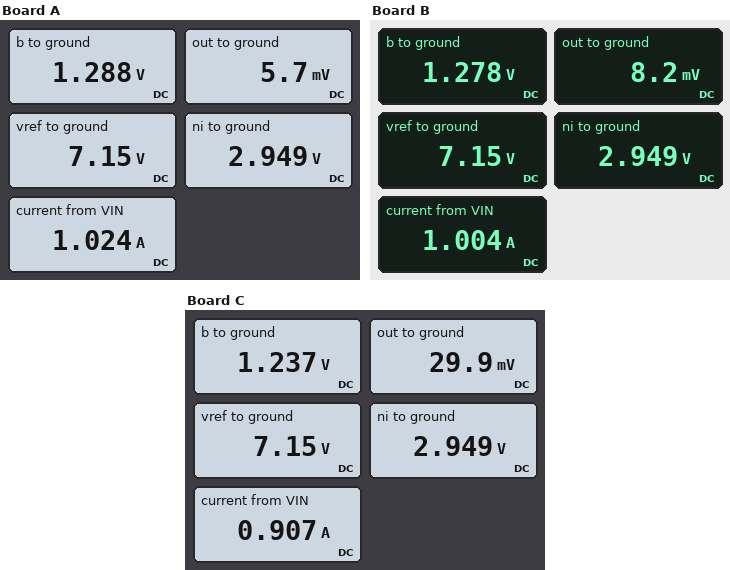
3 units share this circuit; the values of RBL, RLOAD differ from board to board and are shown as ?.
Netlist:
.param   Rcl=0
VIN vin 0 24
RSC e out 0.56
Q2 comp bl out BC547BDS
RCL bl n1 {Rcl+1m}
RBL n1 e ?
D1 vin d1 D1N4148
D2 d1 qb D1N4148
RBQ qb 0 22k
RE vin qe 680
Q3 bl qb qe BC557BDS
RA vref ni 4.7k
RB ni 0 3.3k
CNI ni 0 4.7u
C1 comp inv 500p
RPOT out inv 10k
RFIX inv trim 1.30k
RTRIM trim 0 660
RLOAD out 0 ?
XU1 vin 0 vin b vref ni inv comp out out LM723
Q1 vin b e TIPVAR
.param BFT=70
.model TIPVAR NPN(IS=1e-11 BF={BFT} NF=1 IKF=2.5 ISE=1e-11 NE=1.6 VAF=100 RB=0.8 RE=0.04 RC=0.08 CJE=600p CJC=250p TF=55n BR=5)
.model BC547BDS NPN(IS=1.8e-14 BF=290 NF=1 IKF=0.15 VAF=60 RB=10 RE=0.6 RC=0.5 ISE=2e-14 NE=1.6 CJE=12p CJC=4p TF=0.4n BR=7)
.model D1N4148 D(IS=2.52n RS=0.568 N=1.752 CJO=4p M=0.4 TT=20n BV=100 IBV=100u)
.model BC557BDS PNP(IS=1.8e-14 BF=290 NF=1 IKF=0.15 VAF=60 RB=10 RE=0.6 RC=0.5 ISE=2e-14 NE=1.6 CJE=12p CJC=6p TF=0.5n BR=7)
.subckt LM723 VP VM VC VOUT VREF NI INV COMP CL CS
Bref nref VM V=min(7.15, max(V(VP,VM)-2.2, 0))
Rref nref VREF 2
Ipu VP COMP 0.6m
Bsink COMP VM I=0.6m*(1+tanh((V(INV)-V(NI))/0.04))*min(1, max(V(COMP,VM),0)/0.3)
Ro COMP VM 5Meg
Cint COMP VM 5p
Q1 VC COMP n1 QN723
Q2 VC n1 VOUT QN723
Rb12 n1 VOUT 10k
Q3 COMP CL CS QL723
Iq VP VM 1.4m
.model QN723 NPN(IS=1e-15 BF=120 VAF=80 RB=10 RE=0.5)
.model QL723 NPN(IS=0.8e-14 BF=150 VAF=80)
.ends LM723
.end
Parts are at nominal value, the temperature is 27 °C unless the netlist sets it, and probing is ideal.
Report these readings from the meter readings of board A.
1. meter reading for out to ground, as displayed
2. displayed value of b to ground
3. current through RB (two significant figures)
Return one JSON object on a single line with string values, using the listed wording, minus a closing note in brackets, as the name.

{"meter reading for out to ground, as displayed": "5.7 mV", "displayed value of b to ground": "1.288 V", "current through RB": "890 µA"}
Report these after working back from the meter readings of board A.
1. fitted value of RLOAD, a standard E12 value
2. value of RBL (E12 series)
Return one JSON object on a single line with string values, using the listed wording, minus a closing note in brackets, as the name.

{"fitted value of RLOAD, a standard E12 value": "5.6 mΩ", "value of RBL": "68 Ω"}
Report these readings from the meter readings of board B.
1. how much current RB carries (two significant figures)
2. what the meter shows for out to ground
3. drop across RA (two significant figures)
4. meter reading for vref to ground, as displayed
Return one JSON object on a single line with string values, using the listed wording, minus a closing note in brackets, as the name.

{"how much current RB carries": "890 µA", "what the meter shows for out to ground": "8.2 mV", "drop across RA": "4.2 V", "meter reading for vref to ground, as displayed": "7.15 V"}
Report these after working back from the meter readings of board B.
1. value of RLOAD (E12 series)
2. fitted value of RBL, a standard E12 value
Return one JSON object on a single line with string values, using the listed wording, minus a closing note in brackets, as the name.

{"value of RLOAD": "8.2 mΩ", "fitted value of RBL, a standard E12 value": "82 Ω"}
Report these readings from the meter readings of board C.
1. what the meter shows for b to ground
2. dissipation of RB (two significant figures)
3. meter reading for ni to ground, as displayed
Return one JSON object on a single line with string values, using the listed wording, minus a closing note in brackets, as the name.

{"what the meter shows for b to ground": "1.237 V", "dissipation of RB": "2.6 mW", "meter reading for ni to ground, as displayed": "2.949 V"}
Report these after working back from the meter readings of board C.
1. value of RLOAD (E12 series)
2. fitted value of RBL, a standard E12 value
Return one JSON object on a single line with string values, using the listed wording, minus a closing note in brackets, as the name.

{"value of RLOAD": "0.033 Ω", "fitted value of RBL, a standard E12 value": "150 Ω"}
